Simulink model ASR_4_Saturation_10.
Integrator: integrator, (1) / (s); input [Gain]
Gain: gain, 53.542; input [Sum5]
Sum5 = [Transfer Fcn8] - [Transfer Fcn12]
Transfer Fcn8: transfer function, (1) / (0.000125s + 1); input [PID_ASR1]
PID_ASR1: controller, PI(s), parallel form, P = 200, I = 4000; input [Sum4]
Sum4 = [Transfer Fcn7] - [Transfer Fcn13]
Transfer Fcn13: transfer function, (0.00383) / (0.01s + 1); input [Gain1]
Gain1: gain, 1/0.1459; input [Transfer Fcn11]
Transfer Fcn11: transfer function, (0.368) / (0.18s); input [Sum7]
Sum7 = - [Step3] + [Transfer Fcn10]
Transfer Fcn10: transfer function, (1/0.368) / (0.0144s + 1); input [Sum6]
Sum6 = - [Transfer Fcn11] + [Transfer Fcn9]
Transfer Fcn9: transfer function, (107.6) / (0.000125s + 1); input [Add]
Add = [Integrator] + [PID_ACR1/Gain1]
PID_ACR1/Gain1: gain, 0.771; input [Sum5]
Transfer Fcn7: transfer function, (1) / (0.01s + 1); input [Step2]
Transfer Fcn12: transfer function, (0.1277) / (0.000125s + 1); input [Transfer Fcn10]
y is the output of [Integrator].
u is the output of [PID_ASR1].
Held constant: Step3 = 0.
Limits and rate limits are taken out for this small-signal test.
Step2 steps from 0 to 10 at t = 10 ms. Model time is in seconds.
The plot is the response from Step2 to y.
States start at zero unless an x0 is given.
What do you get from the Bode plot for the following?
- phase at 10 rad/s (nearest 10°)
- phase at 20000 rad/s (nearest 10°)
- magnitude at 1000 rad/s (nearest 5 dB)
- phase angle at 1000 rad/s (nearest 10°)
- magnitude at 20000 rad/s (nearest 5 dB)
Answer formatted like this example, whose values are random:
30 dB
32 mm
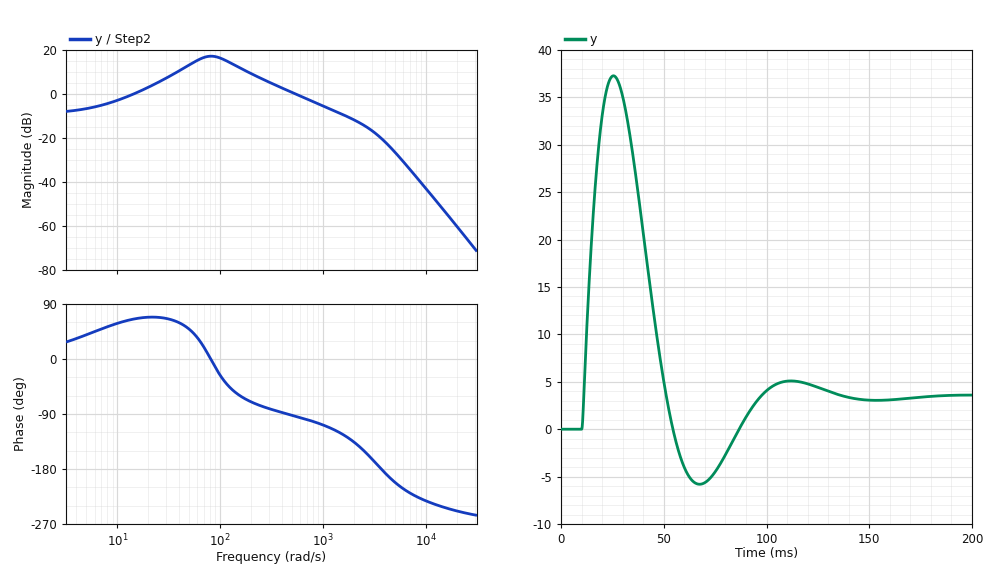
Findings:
60°
-250°
-5 dB
-110°
-60 dB
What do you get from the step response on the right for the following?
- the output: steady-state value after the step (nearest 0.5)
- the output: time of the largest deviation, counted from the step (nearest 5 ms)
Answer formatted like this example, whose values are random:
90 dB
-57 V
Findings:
3.5
15 ms
